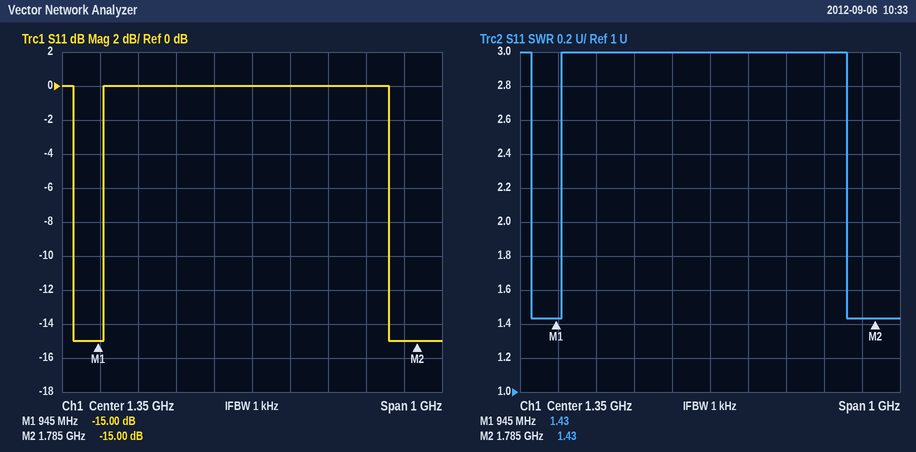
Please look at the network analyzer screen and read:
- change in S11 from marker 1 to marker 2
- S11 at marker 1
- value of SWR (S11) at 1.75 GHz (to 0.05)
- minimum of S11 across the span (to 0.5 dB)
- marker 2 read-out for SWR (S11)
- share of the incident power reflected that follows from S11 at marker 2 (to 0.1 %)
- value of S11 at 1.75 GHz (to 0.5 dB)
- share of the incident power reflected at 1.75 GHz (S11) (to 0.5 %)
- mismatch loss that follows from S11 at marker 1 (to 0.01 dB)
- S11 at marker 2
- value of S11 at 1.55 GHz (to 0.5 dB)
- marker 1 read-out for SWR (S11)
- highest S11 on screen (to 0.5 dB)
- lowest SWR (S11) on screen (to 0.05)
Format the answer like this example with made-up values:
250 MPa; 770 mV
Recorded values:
0.00 dB; -15.00 dB; 1.45; -15.0 dB; 1.43; 3.2 %; -15.0 dB; 3.0 %; 0.14 dB; -15.00 dB; 0.0 dB; 1.43; 0.0 dB; 1.45
